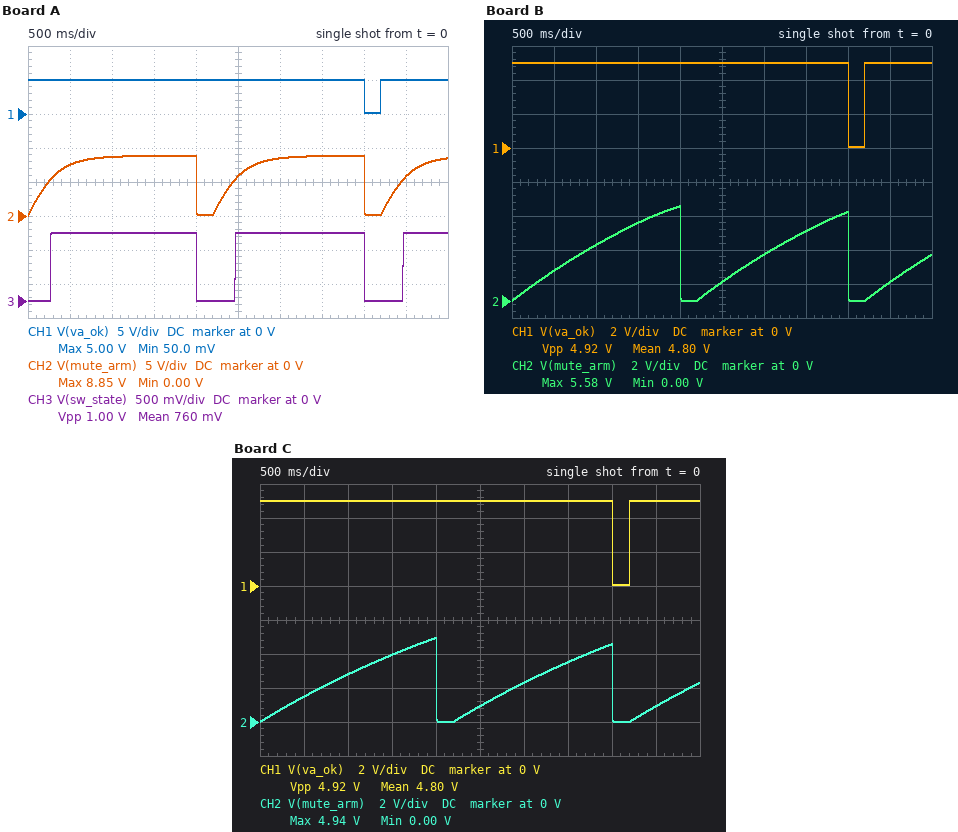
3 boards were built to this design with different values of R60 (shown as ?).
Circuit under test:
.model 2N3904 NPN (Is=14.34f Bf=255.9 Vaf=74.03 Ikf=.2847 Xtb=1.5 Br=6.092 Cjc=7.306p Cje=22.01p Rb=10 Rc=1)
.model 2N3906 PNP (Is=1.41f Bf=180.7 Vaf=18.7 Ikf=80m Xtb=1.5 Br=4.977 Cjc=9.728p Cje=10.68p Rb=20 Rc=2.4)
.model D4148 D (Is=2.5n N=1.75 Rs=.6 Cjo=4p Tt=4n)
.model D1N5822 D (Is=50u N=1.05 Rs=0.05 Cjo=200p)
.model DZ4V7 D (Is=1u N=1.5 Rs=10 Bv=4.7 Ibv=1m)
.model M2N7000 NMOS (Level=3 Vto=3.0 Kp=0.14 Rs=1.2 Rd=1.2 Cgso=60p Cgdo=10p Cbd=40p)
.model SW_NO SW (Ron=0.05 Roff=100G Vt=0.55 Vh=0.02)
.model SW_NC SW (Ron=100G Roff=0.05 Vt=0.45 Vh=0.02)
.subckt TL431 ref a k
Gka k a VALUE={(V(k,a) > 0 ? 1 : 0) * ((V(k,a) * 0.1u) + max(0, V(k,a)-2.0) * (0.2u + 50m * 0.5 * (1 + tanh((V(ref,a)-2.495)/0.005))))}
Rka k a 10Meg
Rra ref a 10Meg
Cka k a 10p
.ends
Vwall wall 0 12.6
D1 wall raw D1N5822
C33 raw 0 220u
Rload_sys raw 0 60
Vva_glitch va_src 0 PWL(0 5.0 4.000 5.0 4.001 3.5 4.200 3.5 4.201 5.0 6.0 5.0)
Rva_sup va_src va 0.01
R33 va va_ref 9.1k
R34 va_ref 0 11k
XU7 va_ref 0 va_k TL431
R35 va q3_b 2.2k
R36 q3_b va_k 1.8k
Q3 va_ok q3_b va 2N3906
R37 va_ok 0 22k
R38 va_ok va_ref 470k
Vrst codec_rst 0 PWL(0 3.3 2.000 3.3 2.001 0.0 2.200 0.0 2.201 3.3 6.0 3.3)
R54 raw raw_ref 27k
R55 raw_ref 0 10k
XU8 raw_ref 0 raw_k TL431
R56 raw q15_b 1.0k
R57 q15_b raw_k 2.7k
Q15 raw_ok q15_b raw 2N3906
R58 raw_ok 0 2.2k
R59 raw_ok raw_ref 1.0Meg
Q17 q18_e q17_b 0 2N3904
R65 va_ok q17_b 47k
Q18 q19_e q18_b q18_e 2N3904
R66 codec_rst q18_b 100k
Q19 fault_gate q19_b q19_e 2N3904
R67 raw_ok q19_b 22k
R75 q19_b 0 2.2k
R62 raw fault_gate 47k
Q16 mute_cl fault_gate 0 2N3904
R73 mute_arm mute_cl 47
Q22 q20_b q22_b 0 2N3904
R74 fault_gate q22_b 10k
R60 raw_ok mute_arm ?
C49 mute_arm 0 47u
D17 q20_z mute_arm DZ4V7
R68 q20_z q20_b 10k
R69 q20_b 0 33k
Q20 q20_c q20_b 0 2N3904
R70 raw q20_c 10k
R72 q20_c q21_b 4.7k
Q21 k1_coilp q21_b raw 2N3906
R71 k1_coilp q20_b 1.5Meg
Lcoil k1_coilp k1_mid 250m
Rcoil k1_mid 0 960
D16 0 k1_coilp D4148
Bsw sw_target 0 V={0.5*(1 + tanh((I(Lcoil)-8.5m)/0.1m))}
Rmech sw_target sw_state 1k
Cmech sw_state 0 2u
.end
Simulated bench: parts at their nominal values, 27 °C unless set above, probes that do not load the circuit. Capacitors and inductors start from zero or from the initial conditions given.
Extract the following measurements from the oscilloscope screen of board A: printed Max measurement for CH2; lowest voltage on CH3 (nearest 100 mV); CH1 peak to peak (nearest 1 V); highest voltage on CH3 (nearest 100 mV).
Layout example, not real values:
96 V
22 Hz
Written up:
8.85 V
0 V
5 V
1.0 V
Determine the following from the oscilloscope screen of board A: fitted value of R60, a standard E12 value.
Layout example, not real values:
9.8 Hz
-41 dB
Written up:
10 kΩ
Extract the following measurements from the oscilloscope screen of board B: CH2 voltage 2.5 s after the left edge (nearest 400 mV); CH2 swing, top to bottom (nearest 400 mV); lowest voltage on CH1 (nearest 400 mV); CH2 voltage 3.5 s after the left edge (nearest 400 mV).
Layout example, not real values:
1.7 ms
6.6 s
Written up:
1.2 V
5.6 V
0 V
4.0 V
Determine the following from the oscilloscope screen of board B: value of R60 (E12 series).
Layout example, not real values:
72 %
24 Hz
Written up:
68 kΩ
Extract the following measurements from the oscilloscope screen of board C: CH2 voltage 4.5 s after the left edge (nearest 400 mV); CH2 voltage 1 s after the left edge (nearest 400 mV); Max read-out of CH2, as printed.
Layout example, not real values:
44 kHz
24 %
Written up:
800 mV
2.8 V
4.94 V
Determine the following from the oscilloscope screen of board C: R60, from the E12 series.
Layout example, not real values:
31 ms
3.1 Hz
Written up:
82 kΩ
